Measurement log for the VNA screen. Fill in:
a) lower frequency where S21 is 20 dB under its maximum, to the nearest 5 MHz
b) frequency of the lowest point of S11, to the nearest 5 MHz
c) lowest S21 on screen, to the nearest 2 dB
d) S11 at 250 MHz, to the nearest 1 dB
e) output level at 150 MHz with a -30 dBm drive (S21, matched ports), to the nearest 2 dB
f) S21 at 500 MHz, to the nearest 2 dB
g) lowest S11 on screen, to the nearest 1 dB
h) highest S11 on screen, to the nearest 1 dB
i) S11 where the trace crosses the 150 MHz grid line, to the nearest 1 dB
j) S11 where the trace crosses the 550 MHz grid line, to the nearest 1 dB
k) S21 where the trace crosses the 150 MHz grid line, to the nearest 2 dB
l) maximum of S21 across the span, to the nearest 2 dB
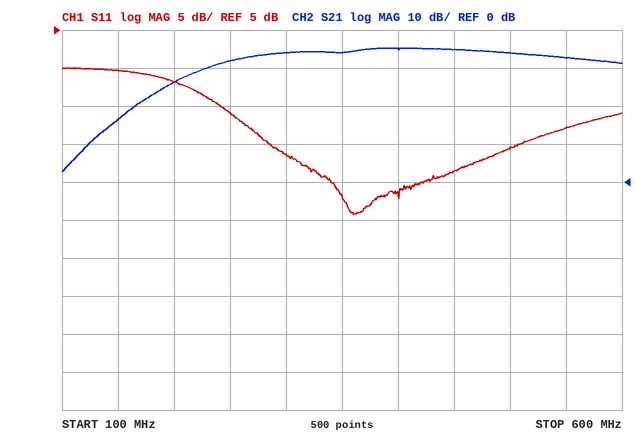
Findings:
145 MHz
360 MHz
2 dB
-6 dB
-14 dBm
34 dB
-19 dB
0 dB
0 dB
-8 dB
16 dB
36 dB
